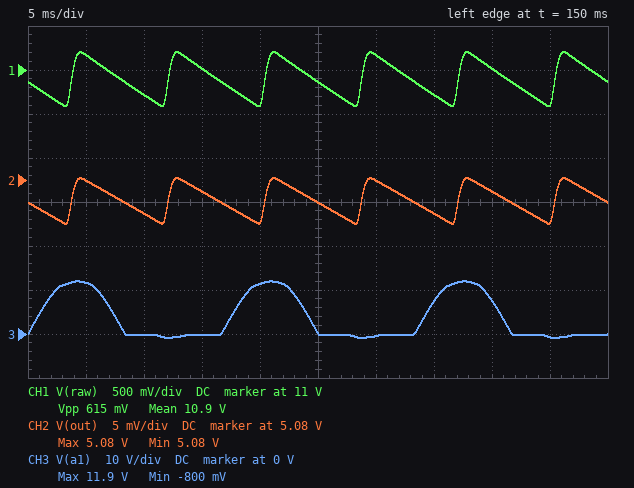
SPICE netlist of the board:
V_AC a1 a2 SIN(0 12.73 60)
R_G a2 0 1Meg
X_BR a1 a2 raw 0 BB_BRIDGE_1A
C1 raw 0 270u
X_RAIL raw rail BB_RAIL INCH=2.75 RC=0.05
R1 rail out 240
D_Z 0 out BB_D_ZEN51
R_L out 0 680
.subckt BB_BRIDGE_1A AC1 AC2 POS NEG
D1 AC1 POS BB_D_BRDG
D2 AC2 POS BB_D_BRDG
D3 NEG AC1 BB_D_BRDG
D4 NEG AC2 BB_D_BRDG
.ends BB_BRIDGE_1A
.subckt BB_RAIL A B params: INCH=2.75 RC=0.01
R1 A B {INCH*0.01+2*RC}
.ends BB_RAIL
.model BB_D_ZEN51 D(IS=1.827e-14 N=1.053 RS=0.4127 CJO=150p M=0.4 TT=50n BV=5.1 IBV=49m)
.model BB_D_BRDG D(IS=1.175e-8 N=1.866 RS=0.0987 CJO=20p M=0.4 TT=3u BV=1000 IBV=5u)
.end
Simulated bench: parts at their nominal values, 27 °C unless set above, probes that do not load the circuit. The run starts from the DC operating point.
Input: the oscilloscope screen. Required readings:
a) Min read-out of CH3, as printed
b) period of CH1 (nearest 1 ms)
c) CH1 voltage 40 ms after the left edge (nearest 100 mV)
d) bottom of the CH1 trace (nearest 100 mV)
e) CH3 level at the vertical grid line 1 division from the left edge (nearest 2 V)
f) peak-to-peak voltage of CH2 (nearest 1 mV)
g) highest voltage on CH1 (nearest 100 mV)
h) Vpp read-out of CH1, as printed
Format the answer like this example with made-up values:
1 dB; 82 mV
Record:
-800 mV; 8 ms; 11.0 V; 10.6 V; 12 V; 5 mV; 11.2 V; 615 mV
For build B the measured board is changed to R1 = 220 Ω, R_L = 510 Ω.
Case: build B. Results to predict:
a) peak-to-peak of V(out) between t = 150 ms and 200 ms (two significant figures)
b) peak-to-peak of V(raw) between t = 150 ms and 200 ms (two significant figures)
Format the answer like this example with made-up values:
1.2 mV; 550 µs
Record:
6.2 mV; 670 mV
